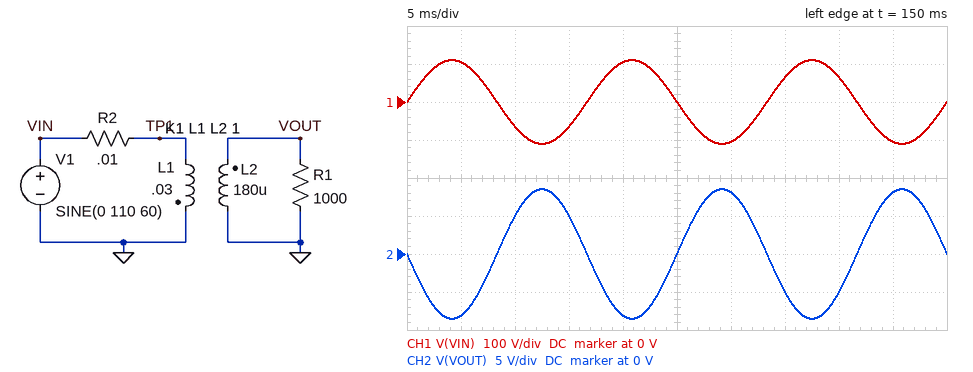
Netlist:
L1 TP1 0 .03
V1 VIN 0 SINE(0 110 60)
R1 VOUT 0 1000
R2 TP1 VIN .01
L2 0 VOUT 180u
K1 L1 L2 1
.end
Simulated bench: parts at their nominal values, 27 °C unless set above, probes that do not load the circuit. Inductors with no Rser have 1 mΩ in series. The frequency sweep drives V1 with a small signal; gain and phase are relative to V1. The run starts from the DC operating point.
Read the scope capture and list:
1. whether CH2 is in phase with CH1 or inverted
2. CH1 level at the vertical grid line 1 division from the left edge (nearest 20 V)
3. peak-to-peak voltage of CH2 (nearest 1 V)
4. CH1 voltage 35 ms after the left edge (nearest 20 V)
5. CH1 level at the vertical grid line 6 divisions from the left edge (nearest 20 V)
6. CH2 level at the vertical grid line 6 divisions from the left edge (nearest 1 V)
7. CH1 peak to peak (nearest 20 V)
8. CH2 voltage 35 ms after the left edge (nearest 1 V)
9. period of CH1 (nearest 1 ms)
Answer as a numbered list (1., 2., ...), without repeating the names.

1. inverted
2. 100 V
3. 17 V
4. 60 V
5. -100 V
6. 8 V
7. 220 V
8. -5 V
9. 17 ms
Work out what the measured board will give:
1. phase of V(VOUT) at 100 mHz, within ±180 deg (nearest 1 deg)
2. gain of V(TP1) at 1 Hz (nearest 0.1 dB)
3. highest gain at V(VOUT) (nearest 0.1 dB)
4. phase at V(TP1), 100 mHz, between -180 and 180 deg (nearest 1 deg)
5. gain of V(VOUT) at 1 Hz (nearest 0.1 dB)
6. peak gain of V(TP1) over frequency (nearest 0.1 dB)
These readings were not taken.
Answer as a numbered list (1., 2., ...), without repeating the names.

1. -150 deg
2. 0 dB
3. -22.2 dB
4. 27 deg
5. -22.2 dB
6. 0 dB
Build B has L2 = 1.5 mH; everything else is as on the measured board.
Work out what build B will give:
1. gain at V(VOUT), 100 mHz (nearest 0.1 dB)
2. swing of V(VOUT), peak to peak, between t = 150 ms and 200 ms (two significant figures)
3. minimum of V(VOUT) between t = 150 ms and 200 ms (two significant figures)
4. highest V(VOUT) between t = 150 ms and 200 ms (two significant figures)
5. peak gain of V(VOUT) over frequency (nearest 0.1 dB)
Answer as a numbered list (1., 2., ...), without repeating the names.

1. -14.3 dB
2. 49 V
3. -25 V
4. 25 V
5. -13.0 dB
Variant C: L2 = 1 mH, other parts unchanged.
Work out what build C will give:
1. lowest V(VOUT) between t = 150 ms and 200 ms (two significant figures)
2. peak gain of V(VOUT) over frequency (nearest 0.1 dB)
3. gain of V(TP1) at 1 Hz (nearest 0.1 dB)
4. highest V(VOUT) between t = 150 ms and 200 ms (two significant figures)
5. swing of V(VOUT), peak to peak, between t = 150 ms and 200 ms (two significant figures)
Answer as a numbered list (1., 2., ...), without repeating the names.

1. -20 V
2. -14.8 dB
3. 0 dB
4. 20 V
5. 40 V
